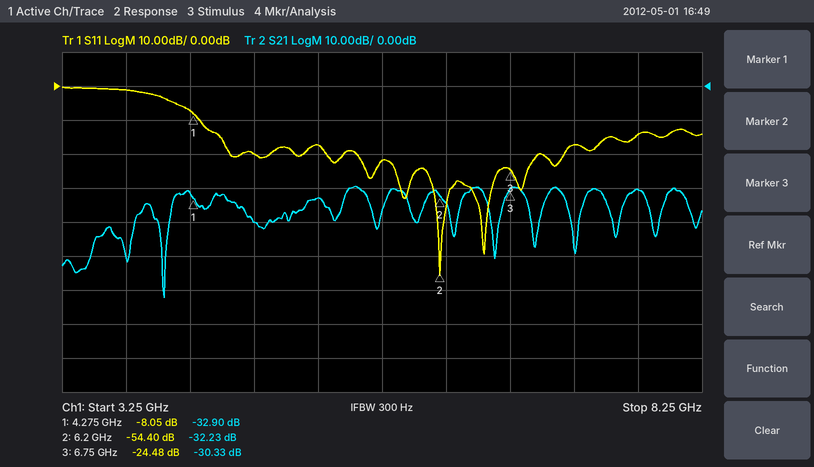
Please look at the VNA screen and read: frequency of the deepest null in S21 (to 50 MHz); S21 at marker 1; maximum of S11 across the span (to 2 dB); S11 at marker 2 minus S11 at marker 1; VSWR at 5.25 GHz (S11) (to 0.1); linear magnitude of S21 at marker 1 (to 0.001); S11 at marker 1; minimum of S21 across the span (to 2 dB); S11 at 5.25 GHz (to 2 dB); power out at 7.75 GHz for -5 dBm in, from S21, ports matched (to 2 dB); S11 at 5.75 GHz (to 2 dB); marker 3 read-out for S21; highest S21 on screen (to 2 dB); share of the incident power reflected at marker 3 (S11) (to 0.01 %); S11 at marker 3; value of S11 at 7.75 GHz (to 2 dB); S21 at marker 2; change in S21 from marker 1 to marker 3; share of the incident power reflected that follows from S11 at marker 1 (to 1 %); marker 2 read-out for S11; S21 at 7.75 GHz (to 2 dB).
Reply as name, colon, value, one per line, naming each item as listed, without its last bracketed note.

frequency of the deepest null in S21: 4.05 GHz
S21 at marker 1: -32.90 dB
maximum of S11 across the span: 0 dB
S11 at marker 2 minus S11 at marker 1: -46.35 dB
VSWR at 5.25 GHz (S11): 1.3
linear magnitude of S21 at marker 1: 0.023
S11 at marker 1: -8.05 dB
minimum of S21 across the span: -62 dB
S11 at 5.25 GHz: -18 dB
power out at 7.75 GHz for -5 dBm in, from S21, ports matched: -36 dBm
S11 at 5.75 GHz: -22 dB
marker 3 read-out for S21: -30.33 dB
highest S21 on screen: -30 dB
share of the incident power reflected at marker 3 (S11): 0.36 %
S11 at marker 3: -24.48 dB
value of S11 at 7.75 GHz: -14 dB
S21 at marker 2: -32.23 dB
change in S21 from marker 1 to marker 3: 2.57 dB
share of the incident power reflected that follows from S11 at marker 1: 16 %
marker 2 read-out for S11: -54.40 dB
S21 at 7.75 GHz: -30 dB
